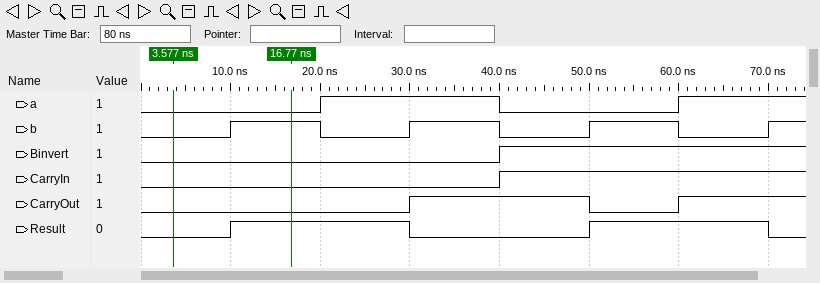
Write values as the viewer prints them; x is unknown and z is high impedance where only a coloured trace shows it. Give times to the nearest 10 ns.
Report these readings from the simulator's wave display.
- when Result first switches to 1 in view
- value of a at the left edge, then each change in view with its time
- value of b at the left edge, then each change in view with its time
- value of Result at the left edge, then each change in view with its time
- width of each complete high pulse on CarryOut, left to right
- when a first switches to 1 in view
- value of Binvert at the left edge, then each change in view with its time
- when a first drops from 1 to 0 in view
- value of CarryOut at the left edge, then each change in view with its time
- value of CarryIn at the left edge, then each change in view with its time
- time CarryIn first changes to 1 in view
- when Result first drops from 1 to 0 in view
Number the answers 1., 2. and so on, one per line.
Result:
1. 10 ns
2. 0, 1 at 20 ns, 0 at 40 ns, 1 at 60 ns
3. 0, 1 at 10 ns, 0 at 20 ns, 1 at 30 ns, 0 at 40 ns, 1 at 50 ns, 0 at 60 ns, 1 at 70 ns
4. 0, 1 at 10 ns, 0 at 30 ns, 1 at 50 ns, 0 at 70 ns
5. 20 ns
6. 20 ns
7. 0, 1 at 40 ns
8. 40 ns
9. 0, 1 at 30 ns, 0 at 50 ns, 1 at 60 ns
10. 0, 1 at 40 ns
11. 40 ns
12. 30 ns
